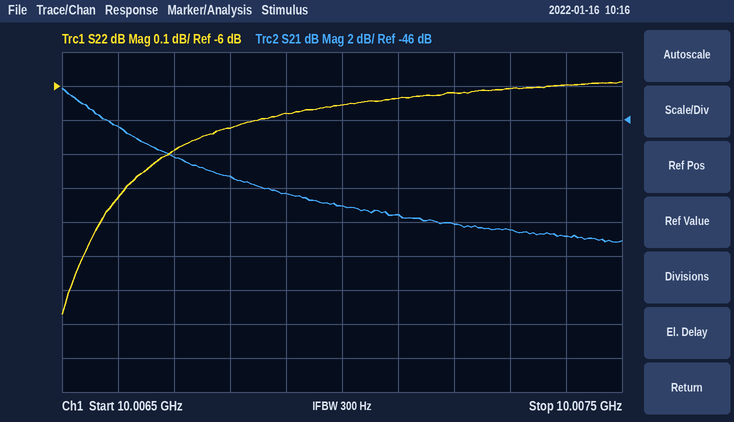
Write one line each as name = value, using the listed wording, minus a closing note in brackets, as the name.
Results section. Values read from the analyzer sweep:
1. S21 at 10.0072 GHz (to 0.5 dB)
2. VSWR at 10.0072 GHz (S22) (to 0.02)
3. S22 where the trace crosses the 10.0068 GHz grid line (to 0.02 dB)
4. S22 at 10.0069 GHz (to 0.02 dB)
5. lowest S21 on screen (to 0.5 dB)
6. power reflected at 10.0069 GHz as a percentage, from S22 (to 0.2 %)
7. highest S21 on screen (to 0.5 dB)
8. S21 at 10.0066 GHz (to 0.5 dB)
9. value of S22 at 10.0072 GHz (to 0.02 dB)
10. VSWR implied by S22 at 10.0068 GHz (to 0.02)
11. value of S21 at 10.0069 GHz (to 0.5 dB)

S21 at 10.0072 GHz = -52.0 dB
VSWR at 10.0072 GHz (S22) = 3.00
S22 where the trace crosses the 10.0068 GHz grid line = -6.12 dB
S22 at 10.0069 GHz = -6.08 dB
lowest S21 on screen = -53.0 dB
power reflected at 10.0069 GHz as a percentage, from S22 = 24.6 %
highest S21 on screen = -44.0 dB
S21 at 10.0066 GHz = -46.5 dB
value of S22 at 10.0072 GHz = -6.02 dB
VSWR implied by S22 at 10.0068 GHz = 2.96
value of S21 at 10.0069 GHz = -50.5 dB
